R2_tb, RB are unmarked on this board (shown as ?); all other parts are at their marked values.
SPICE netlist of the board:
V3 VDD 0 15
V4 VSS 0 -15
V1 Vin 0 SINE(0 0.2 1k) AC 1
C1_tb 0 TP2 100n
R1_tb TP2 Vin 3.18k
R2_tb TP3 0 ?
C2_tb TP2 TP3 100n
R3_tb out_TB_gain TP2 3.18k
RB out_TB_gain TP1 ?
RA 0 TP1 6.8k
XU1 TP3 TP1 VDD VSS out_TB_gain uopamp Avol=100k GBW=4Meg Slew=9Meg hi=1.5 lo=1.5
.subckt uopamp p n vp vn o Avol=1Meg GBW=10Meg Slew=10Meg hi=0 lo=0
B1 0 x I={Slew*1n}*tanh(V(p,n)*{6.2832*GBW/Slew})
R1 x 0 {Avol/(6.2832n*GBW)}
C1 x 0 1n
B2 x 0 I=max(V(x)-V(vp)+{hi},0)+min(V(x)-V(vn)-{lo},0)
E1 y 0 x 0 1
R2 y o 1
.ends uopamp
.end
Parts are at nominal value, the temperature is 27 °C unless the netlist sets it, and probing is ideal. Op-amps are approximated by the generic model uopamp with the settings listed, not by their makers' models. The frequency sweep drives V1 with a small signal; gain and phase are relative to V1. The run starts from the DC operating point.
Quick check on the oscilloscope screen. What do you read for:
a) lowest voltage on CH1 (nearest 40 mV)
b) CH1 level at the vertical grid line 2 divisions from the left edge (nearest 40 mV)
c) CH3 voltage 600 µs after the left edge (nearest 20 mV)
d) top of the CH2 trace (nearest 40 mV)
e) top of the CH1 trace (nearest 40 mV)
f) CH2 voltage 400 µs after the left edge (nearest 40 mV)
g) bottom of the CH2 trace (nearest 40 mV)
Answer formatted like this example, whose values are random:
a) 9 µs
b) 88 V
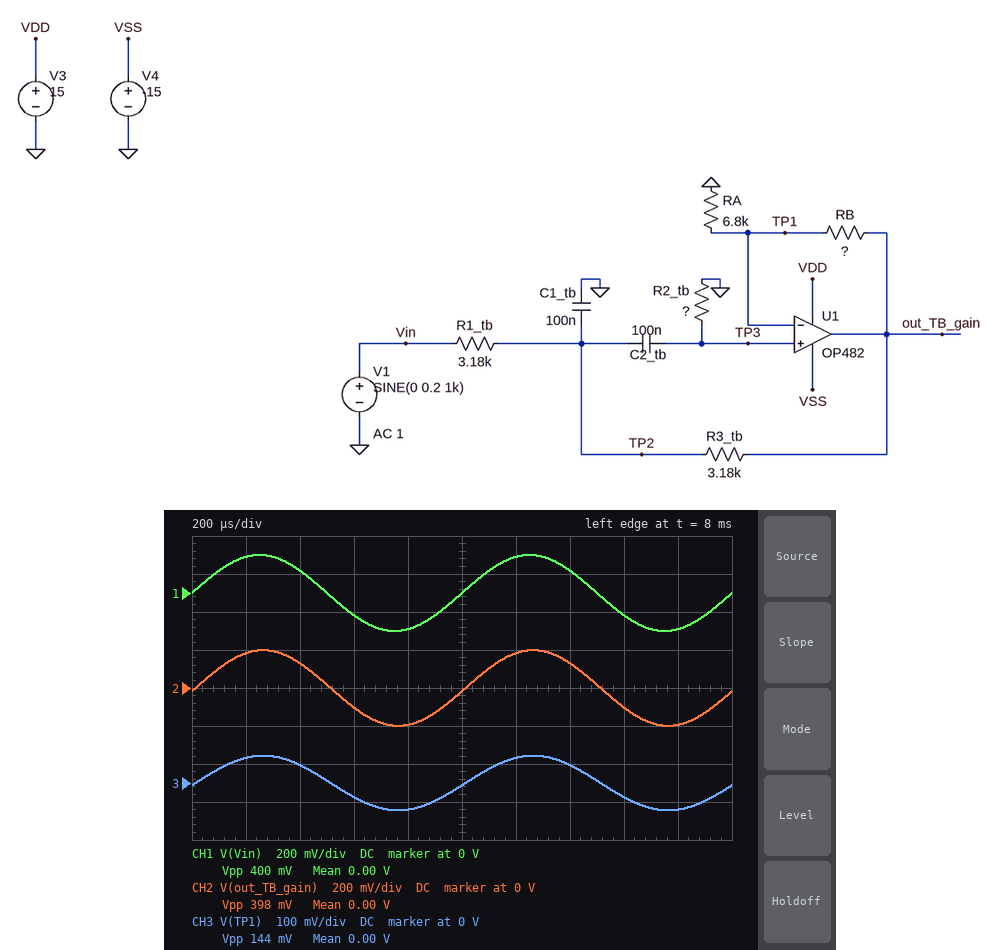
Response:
a) -200 mV
b) 120 mV
c) -40 mV
d) 200 mV
e) 200 mV
f) 120 mV
g) -200 mV
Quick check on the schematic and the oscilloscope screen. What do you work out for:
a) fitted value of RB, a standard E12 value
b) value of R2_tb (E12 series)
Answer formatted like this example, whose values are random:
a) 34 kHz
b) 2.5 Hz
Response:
a) 12 kΩ
b) 1.8 kΩ
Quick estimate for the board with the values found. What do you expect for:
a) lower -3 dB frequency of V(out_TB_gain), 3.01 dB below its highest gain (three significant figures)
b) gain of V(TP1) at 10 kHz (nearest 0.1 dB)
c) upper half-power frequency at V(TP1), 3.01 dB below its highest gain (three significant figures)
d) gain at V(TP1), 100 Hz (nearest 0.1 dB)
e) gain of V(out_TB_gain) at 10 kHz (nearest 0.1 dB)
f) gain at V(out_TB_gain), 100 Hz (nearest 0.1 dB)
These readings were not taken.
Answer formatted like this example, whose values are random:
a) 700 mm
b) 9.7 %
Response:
a) 475 Hz
b) -26.0 dB
c) 1.86 kHz
d) -25.0 dB
e) -17.2 dB
f) -16.1 dB
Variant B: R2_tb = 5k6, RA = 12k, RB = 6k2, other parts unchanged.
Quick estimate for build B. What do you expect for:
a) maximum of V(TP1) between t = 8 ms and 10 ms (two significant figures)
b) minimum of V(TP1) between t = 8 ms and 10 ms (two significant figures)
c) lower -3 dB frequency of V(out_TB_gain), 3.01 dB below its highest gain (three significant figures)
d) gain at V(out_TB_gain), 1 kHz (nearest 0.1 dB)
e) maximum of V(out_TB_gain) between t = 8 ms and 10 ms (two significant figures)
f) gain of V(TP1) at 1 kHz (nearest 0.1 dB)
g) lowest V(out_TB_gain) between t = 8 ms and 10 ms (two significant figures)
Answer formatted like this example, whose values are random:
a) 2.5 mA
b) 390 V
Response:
a) 93 mV
b) -93 mV
c) 265 Hz
d) -3.1 dB
e) 140 mV
f) -6.7 dB
g) -140 mV
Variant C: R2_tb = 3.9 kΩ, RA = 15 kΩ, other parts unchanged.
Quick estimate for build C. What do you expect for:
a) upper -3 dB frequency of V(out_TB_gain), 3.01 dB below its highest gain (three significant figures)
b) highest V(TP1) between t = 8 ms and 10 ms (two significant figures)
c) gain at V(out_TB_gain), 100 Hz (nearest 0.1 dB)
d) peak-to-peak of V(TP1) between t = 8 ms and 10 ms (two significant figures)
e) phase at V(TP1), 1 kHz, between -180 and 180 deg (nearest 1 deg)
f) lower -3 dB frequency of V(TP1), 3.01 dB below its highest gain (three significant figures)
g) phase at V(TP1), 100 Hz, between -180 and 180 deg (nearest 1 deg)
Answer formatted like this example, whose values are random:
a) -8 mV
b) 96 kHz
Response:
a) 1.24 kHz
b) 92 mV
c) -13.1 dB
d) 180 mV
e) -33 deg
f) 328 Hz
g) 77 deg
